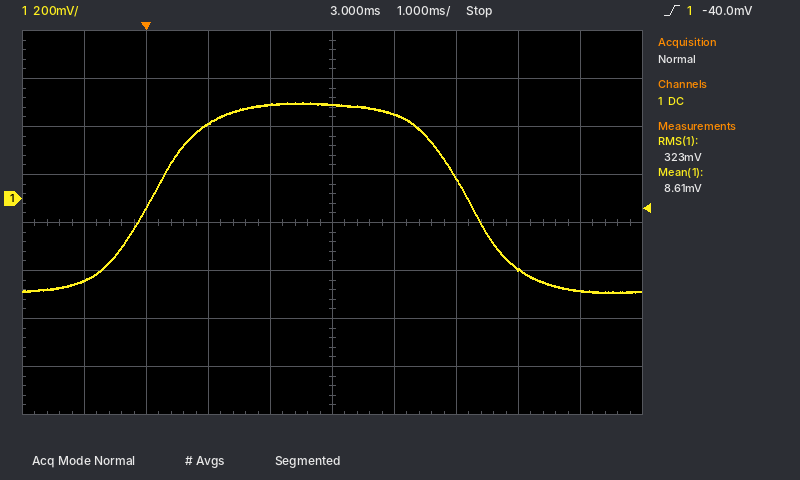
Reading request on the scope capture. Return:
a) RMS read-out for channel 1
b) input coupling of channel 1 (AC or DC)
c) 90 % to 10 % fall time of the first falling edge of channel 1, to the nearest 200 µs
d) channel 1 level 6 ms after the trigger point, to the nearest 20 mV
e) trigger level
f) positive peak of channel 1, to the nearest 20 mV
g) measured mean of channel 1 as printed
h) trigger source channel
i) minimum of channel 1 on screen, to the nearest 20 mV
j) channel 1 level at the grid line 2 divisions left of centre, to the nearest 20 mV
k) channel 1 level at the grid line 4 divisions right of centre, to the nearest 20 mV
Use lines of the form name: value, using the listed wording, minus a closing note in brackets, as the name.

RMS read-out for channel 1: 323 mV
input coupling of channel 1: DC
90 % to 10 % fall time of the first falling edge of channel 1, to the nearest 200 µs: 1.8 ms
channel 1 level 6 ms after the trigger point, to the nearest 20 mV: -300 mV
trigger level: -40.0 mV
positive peak of channel 1, to the nearest 20 mV: 400 mV
measured mean of channel 1 as printed: 8.61 mV
trigger source channel: channel 1
minimum of channel 1 on screen, to the nearest 20 mV: -400 mV
channel 1 level at the grid line 2 divisions left of centre, to the nearest 20 mV: 320 mV
channel 1 level at the grid line 4 divisions right of centre, to the nearest 20 mV: -380 mV
